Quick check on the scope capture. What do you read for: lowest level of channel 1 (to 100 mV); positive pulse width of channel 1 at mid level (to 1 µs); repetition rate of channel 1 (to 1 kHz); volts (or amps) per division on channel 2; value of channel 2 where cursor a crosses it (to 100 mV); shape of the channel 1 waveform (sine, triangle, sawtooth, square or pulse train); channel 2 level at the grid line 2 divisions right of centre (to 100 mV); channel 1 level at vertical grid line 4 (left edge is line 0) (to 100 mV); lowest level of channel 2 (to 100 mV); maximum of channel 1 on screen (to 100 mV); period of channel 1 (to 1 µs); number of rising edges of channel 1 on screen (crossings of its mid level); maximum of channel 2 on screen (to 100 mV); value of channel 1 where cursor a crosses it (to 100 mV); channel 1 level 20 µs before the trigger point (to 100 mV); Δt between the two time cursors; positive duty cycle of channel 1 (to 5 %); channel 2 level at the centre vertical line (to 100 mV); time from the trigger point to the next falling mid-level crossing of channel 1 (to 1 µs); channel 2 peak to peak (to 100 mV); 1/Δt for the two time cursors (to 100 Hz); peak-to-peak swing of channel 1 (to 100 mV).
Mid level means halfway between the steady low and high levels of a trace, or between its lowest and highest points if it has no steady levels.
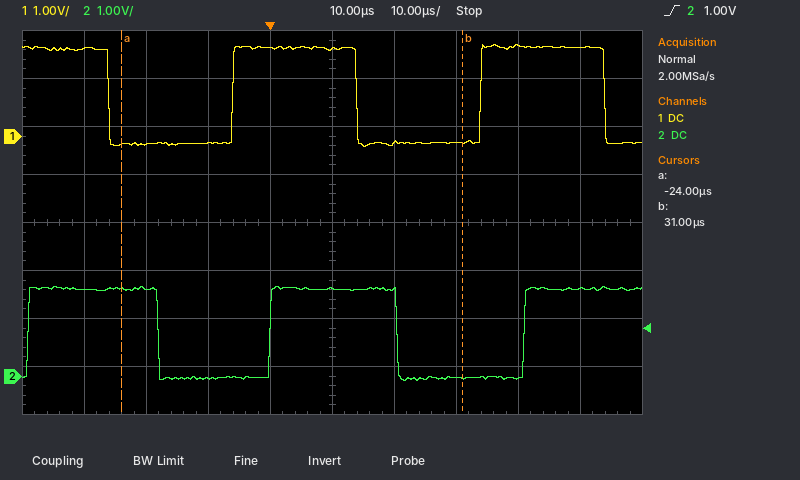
-200 mV
20 µs
25 kHz
1 V
1.8 V
square
0.0 V
1.8 V
-100 mV
1.9 V
40 µs
2
1.9 V
-200 mV
-200 mV
55 µs
50 %
1.8 V
14 µs
2.0 V
18.2 kHz
2.1 V
